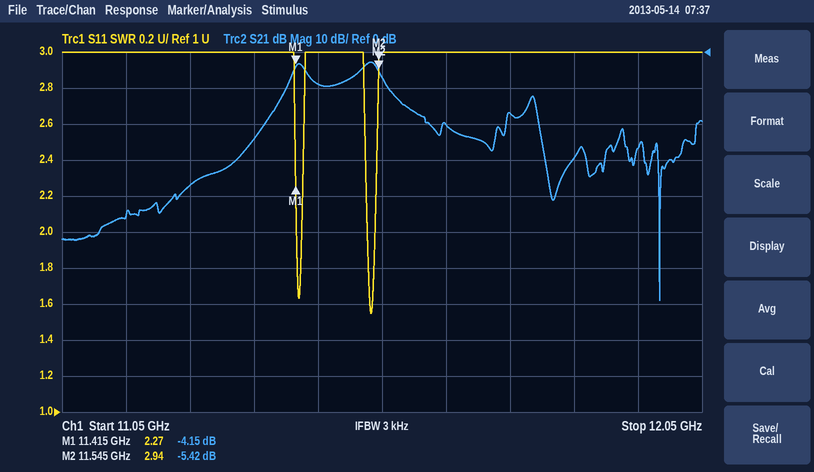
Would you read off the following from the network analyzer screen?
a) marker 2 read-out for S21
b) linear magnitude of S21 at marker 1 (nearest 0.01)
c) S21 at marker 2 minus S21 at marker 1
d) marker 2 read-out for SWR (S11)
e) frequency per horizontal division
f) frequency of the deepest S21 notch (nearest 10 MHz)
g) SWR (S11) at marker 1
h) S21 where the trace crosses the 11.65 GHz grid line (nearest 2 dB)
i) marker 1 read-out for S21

-5.42 dB
0.62
-1.27 dB
2.94
100 MHz
11.98 GHz
2.27
-20 dB
-4.15 dB
